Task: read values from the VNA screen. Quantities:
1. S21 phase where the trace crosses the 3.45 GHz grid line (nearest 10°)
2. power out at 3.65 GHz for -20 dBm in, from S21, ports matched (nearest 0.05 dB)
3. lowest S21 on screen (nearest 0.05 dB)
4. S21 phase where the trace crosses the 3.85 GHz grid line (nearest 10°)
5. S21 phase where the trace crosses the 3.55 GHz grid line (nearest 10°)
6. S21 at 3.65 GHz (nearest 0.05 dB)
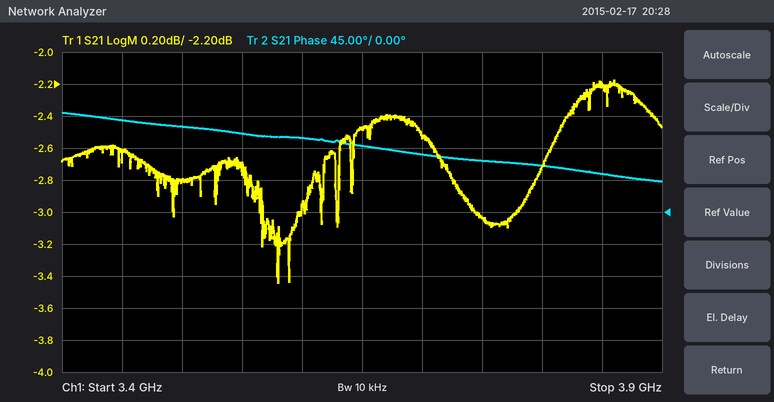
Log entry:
130°
-22.50 dBm
-3.45 dB
50°
110°
-2.50 dB
